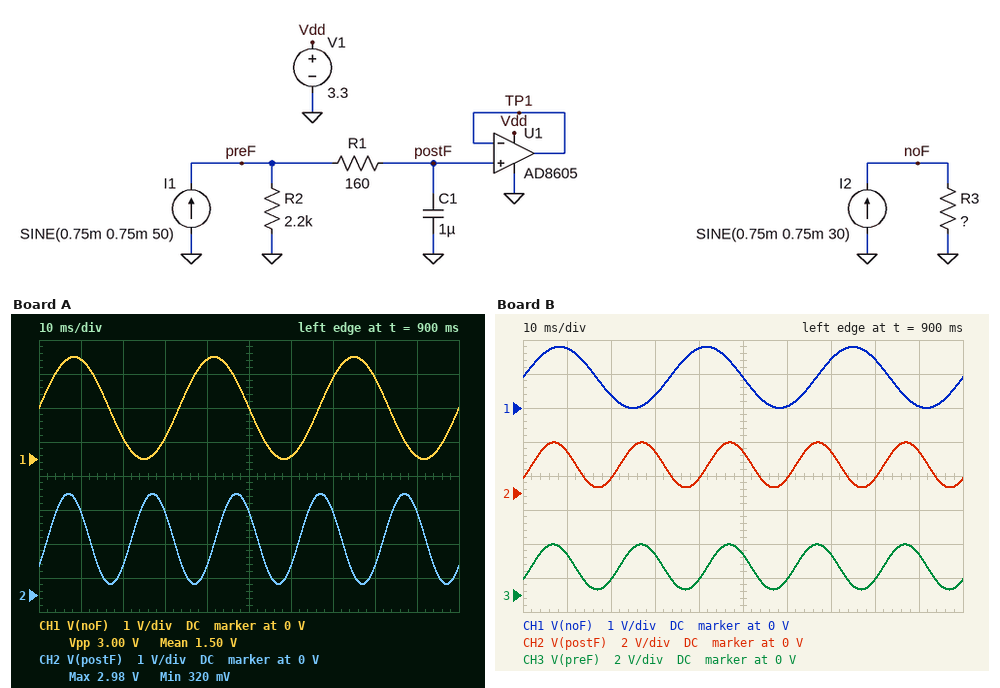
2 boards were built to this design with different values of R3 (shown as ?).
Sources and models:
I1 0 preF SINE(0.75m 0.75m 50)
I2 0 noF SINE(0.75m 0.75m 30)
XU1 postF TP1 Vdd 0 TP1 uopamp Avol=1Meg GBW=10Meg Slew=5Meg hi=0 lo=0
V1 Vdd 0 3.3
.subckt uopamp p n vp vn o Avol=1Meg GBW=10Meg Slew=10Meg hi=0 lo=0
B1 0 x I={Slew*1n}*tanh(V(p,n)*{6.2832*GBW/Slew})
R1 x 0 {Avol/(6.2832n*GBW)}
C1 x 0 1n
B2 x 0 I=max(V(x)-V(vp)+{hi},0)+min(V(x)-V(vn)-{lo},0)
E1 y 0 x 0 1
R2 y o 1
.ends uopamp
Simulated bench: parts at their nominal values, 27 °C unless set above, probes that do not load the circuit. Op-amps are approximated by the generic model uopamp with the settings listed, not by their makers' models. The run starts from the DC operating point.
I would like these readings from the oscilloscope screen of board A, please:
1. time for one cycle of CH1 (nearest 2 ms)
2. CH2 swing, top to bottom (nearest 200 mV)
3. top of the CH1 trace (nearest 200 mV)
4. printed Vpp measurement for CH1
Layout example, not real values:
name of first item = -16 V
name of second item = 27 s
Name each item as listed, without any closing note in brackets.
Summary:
time for one cycle of CH1 = 34 ms
CH2 swing, top to bottom = 2.6 V
top of the CH1 trace = 3.0 V
printed Vpp measurement for CH1 = 3.00 V
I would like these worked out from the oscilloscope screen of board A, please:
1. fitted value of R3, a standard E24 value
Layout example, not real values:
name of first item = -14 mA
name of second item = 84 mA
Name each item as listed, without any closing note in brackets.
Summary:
fitted value of R3, a standard E24 value = 2 kΩ
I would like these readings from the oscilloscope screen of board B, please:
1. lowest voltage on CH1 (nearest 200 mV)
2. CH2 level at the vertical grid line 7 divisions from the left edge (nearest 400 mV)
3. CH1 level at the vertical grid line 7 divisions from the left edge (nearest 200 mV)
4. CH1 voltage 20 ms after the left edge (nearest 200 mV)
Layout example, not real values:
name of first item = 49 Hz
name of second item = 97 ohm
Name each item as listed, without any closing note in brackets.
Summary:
lowest voltage on CH1 = 0 V
CH2 level at the vertical grid line 7 divisions from the left edge = 2.4 V
CH1 level at the vertical grid line 7 divisions from the left edge = 1.4 V
CH1 voltage 20 ms after the left edge = 400 mV
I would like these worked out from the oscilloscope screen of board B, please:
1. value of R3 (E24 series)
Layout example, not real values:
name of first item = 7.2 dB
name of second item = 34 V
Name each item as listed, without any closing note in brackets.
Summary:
value of R3 = 1.2 kΩ
